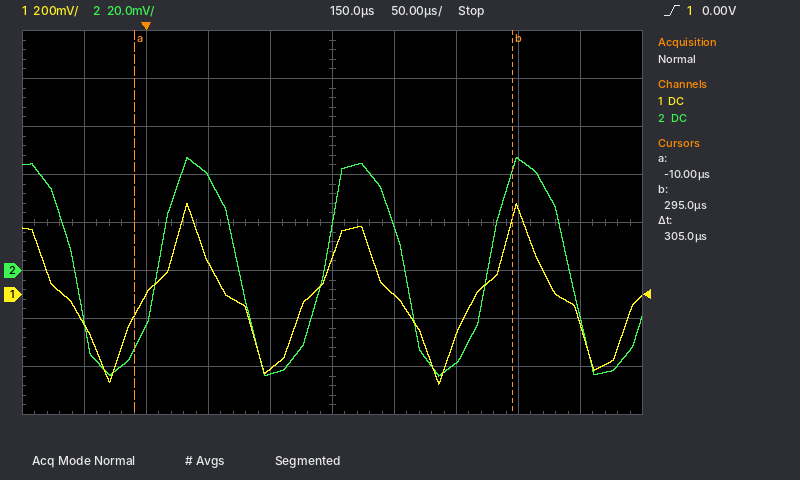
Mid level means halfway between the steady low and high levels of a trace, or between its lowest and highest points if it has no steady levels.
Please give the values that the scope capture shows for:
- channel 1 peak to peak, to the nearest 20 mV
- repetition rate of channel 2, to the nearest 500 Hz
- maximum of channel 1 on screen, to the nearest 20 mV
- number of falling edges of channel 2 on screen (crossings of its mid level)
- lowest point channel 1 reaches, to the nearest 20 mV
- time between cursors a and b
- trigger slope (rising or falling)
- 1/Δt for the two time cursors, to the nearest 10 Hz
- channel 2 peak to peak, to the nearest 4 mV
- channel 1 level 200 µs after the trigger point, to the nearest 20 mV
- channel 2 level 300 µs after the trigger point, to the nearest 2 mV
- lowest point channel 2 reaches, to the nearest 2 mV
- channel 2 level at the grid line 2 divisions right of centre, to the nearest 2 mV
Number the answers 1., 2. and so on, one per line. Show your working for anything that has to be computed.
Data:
1. 380 mV − (-380 mV) = 760 mV
2. 7.5 kHz
3. 380 mV
4. 4
5. -380 mV
6. 305 µs
7. rising
8. 1 / 305 µs ≈ 3.28 kHz
9. 92 mV
10. 0 mV
11. 46 mV
12. -44 mV
13. -38 mV
